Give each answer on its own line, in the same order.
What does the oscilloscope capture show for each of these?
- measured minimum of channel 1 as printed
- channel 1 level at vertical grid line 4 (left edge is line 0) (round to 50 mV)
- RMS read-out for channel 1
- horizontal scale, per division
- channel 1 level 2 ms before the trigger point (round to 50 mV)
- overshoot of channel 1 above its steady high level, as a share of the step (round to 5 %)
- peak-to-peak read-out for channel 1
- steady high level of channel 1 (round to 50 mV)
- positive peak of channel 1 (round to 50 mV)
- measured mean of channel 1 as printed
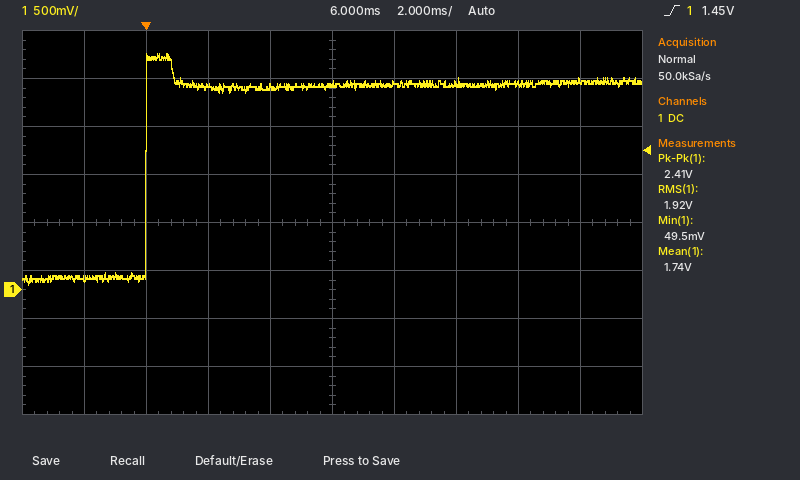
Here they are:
49.5 mV
2.10 V
1.92 V
2 ms
100 mV
15 %
2.41 V
2.15 V
2.45 V
1.74 V
